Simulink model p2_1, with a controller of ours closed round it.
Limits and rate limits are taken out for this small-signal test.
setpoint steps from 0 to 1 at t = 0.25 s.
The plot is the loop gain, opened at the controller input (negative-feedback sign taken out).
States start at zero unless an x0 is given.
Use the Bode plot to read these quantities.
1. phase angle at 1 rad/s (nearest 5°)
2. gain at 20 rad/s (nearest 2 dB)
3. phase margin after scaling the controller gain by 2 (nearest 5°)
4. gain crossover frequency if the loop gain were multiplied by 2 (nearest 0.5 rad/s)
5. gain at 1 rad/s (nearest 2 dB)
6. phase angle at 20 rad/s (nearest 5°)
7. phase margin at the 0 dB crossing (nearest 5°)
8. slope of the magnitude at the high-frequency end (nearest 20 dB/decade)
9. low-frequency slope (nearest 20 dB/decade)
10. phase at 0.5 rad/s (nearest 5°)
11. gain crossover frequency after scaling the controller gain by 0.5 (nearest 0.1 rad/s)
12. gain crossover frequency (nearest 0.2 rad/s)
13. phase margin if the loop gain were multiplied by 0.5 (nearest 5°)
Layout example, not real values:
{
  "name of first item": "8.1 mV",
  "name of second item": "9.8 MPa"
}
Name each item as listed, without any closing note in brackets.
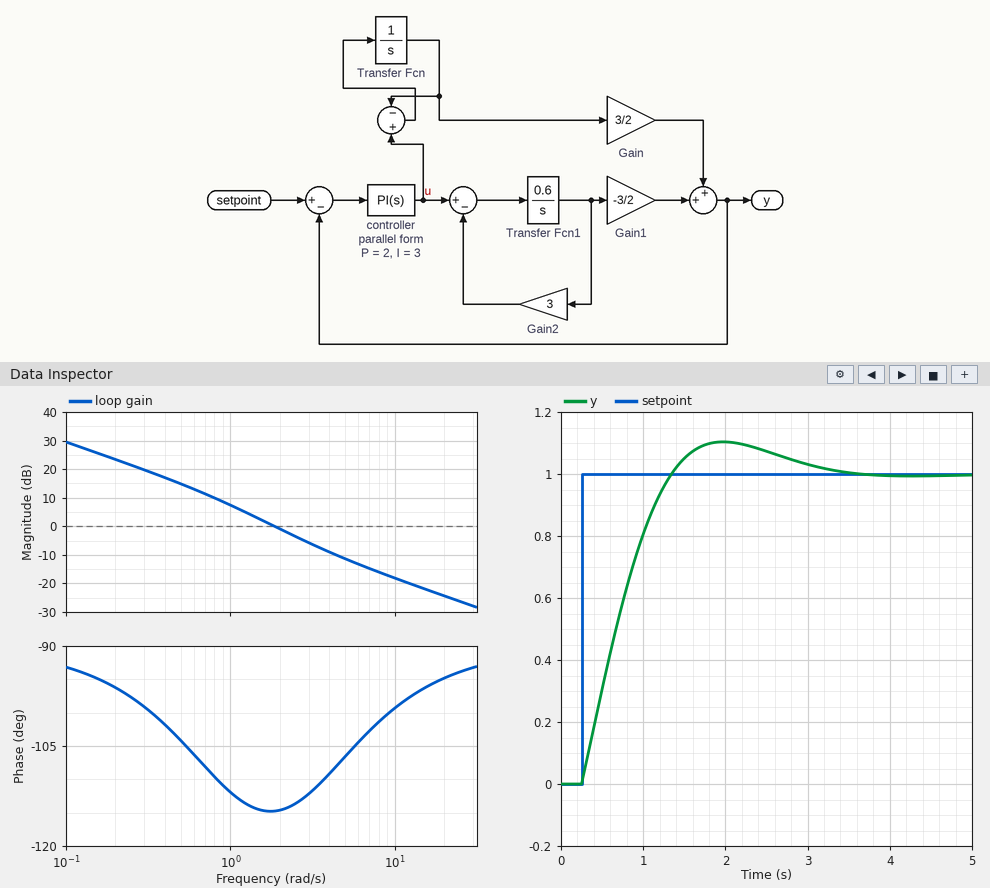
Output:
{
  "phase angle at 1 rad/s": "-110°",
  "gain at 20 rad/s": "-24 dB",
  "phase margin after scaling the controller gain by 2": "70°",
  "gain crossover frequency if the loop gain were multiplied by 2": "3.0 rad/s",
  "gain at 1 rad/s": "8 dB",
  "phase angle at 20 rad/s": "-95°",
  "phase margin at the 0 dB crossing": "65°",
  "slope of the magnitude at the high-frequency end": "-20 dB/decade",
  "low-frequency slope": "-20 dB/decade",
  "phase at 0.5 rad/s": "-105°",
  "gain crossover frequency after scaling the controller gain by 0.5": "1.1 rad/s",
  "gain crossover frequency": "1.8 rad/s",
  "phase margin if the loop gain were multiplied by 0.5": "65°"
}
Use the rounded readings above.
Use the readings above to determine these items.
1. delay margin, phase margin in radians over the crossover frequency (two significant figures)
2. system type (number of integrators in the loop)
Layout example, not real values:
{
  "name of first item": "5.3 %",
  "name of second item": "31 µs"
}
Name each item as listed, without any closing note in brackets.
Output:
{
  "delay margin, phase margin in radians over the crossover frequency": "0.63 s",
  "system type": "1"
}
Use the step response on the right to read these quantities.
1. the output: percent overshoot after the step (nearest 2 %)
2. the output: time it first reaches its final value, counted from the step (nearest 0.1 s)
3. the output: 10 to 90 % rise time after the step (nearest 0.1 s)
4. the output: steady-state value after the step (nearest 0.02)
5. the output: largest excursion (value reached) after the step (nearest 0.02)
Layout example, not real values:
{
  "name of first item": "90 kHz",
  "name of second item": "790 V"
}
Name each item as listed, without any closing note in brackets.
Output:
{
  "the output: percent overshoot after the step": "10 %",
  "the output: time it first reaches its final value, counted from the step": "1.1 s",
  "the output: 10 to 90 % rise time after the step": "0.8 s",
  "the output: steady-state value after the step": "1.00",
  "the output: largest excursion (value reached) after the step": "1.10"
}
